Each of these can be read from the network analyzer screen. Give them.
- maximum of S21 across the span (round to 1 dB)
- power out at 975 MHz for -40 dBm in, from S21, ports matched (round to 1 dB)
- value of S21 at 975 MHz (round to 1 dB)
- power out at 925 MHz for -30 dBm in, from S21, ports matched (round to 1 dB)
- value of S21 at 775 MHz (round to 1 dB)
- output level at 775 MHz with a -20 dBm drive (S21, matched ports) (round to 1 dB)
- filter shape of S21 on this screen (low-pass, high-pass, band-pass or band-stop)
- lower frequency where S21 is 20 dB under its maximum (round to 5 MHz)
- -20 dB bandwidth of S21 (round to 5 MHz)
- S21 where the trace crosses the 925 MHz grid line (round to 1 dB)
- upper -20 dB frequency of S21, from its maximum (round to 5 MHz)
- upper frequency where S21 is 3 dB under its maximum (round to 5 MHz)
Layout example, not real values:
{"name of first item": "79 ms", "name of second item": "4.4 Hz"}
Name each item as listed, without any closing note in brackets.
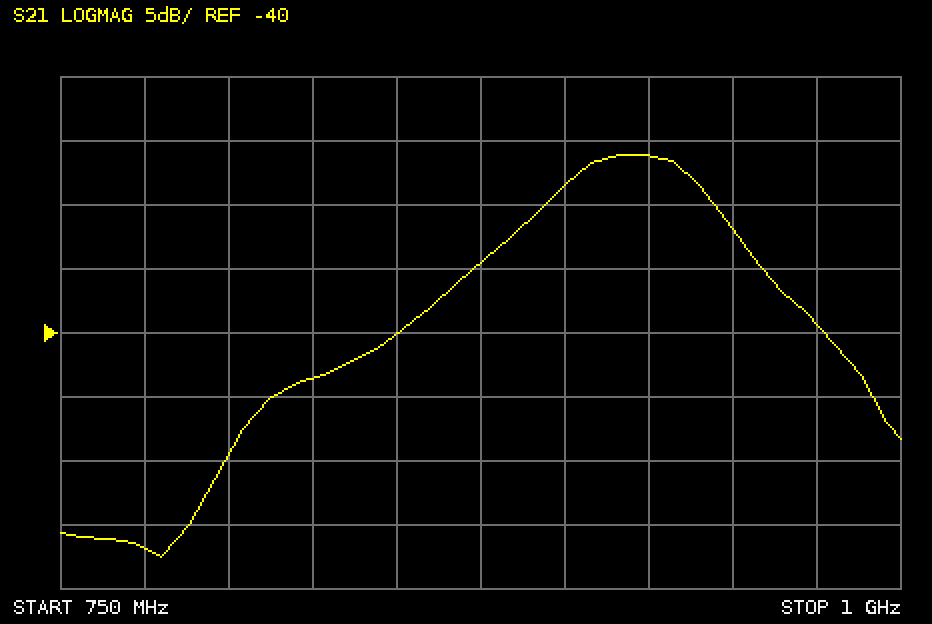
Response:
{"maximum of S21 across the span": "-26 dB", "power out at 975 MHz for -40 dBm in, from S21, ports matched": "-79 dBm", "value of S21 at 975 MHz": "-39 dB", "power out at 925 MHz for -30 dBm in, from S21, ports matched": "-56 dBm", "value of S21 at 775 MHz": "-57 dB", "output level at 775 MHz with a -20 dBm drive (S21, matched ports)": "-77 dBm", "filter shape of S21 on this screen": "band-pass", "lower frequency where S21 is 20 dB under its maximum": "810 MHz", "-20 dB bandwidth of S21": "185 MHz", "S21 where the trace crosses the 925 MHz grid line": "-26 dB", "upper -20 dB frequency of S21, from its maximum": "995 MHz", "upper frequency where S21 is 3 dB under its maximum": "940 MHz"}
